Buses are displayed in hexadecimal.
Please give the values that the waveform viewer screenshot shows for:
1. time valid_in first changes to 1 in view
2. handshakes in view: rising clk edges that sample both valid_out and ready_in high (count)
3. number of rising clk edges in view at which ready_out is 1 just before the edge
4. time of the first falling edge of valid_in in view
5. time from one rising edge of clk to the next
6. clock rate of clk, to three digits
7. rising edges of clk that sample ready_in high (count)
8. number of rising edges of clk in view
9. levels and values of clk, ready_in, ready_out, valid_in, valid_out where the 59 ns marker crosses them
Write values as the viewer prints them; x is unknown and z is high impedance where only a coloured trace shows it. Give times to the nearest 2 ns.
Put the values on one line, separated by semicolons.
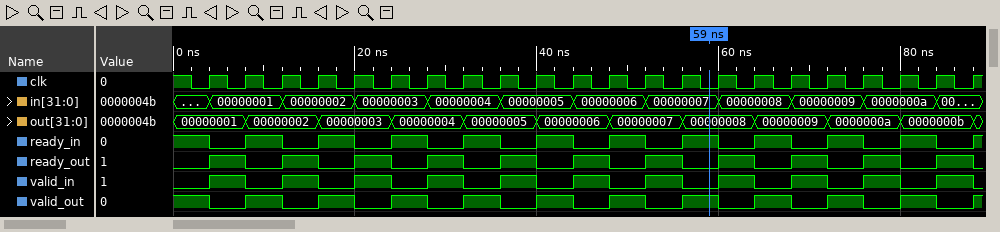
4 ns; 11; 11; 8 ns; 4 ns; 250 MHz; 11; 22; clk=0, ready_in=1, ready_out=0, valid_in=0, valid_out=1
